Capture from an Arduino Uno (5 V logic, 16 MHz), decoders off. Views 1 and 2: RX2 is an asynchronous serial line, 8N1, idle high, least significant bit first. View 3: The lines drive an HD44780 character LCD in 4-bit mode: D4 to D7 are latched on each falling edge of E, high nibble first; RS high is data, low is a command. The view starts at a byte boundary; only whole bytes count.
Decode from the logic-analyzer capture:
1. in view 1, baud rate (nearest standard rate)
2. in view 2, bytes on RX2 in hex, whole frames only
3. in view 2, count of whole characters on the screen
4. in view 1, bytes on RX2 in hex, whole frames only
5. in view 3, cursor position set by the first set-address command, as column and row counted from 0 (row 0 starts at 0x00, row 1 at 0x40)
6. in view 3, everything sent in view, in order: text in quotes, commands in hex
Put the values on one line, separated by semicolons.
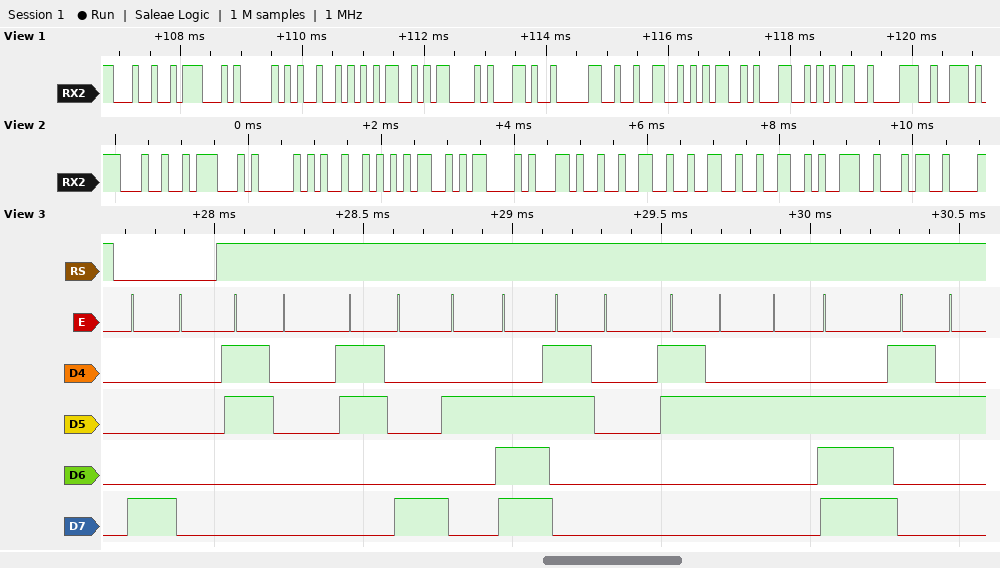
9600 baud; 24 47 50 52 4D 43 2C 32 32 32 39 34; 12; 24 47 50 52 4D 43 2C 30 32 35 31 35 38; column 0, row 0; 0x80 "08.02.2"
